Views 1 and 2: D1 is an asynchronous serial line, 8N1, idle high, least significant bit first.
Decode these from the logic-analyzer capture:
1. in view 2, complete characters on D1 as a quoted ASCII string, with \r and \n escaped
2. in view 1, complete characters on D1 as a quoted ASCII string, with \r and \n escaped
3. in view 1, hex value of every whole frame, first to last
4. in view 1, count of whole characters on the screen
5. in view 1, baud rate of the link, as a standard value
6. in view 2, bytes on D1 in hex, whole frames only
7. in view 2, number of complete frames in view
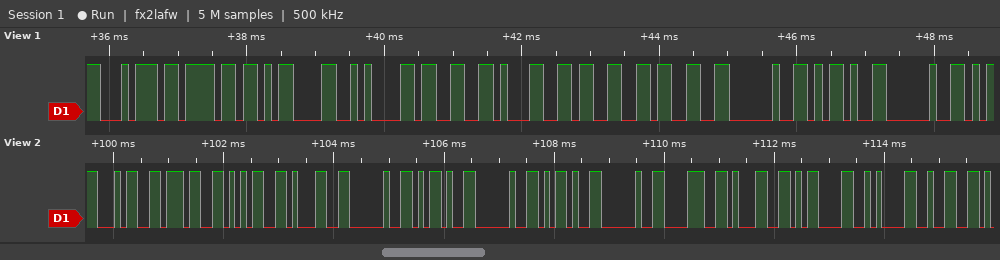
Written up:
"4751 - - 81\r\n2"
"to\r\n3133 - "
74 6F 0D 0A 33 31 33 33 20 2D 20
11
9600 baud
34 37 35 31 20 2D 20 2D 20 38 31 0D 0A 32
14
